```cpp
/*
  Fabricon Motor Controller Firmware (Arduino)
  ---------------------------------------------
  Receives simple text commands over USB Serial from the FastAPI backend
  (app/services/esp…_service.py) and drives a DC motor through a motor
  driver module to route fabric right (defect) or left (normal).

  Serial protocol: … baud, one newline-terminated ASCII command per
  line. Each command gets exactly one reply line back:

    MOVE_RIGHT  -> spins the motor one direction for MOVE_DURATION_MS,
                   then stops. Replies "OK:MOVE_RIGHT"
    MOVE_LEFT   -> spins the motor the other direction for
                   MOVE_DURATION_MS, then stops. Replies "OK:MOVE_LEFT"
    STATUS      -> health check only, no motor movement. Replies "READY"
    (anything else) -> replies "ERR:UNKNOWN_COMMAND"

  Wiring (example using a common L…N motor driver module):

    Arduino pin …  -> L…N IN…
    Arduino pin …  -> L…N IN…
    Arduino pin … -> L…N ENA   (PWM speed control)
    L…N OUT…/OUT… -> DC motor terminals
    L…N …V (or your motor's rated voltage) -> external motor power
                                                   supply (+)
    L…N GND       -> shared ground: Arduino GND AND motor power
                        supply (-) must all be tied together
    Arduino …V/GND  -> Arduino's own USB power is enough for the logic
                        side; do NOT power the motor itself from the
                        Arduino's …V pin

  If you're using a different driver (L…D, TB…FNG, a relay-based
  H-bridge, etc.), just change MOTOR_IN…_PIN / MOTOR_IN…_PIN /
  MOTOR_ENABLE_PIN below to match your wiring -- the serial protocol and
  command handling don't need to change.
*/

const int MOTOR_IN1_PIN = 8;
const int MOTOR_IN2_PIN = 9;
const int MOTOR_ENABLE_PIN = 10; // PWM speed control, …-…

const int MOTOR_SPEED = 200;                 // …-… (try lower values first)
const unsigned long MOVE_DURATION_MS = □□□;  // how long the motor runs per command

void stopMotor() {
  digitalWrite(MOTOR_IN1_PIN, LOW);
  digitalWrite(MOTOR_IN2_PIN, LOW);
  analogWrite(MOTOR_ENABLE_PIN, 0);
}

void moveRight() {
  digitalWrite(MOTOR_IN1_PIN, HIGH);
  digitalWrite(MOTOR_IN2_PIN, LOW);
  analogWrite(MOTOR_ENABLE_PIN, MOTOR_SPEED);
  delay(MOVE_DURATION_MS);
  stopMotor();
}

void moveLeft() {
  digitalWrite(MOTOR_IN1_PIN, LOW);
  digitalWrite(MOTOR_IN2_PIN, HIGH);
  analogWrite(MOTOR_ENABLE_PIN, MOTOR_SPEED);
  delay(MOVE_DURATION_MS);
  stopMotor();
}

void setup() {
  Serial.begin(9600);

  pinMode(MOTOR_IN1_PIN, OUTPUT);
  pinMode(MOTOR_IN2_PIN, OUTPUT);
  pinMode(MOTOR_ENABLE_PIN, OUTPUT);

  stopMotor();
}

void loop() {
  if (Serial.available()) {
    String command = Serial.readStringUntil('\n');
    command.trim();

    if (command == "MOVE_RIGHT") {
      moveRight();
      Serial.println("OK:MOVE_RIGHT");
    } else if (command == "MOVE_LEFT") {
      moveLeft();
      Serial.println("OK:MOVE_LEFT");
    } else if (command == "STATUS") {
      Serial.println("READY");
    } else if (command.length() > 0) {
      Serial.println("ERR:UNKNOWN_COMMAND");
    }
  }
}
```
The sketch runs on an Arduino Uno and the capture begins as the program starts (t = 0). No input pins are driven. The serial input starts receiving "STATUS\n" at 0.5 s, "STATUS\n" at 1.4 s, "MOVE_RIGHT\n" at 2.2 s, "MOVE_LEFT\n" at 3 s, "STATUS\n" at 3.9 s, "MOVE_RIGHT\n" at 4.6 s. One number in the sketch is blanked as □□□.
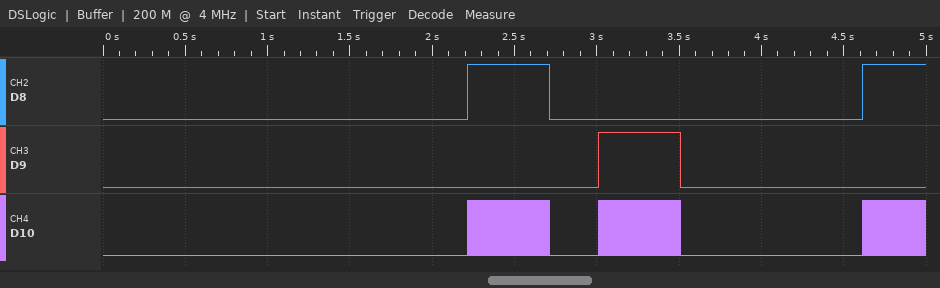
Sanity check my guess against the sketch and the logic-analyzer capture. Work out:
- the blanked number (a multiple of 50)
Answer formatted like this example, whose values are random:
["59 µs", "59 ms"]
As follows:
["500"]
